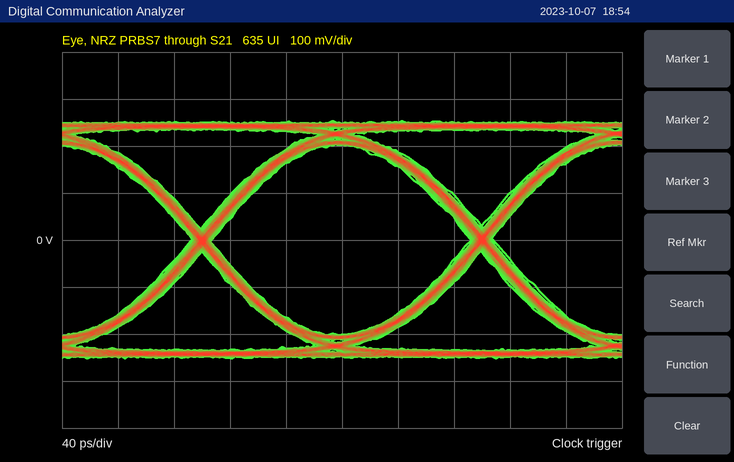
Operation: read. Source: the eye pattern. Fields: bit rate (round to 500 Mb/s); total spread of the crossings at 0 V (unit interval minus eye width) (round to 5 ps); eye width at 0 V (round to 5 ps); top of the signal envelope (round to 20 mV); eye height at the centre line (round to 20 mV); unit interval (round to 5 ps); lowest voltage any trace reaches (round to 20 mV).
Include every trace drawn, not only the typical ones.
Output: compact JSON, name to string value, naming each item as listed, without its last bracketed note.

{"bit rate": "5.0 Gb/s", "total spread of the crossings at 0 V (unit interval minus eye width)": "15 ps", "eye width at 0 V": "185 ps", "top of the signal envelope": "260 mV", "eye height at the centre line": "400 mV", "unit interval": "200 ps", "lowest voltage any trace reaches": "-260 mV"}
